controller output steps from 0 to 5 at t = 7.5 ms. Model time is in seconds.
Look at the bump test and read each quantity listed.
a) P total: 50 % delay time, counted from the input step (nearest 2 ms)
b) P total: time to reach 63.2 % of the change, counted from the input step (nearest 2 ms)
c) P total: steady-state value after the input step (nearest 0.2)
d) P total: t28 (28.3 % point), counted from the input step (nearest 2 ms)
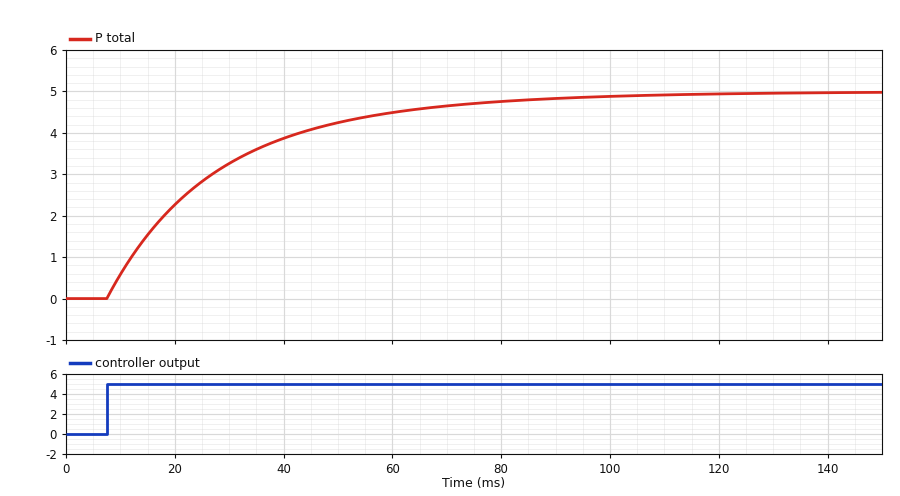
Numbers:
14 ms
22 ms
5.0
6 ms
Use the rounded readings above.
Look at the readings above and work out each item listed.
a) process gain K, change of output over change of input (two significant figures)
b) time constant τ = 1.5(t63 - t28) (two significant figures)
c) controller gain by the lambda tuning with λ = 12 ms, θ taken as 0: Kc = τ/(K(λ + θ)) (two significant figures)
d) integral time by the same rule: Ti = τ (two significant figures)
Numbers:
1.0
24 ms
2.0
24 ms
